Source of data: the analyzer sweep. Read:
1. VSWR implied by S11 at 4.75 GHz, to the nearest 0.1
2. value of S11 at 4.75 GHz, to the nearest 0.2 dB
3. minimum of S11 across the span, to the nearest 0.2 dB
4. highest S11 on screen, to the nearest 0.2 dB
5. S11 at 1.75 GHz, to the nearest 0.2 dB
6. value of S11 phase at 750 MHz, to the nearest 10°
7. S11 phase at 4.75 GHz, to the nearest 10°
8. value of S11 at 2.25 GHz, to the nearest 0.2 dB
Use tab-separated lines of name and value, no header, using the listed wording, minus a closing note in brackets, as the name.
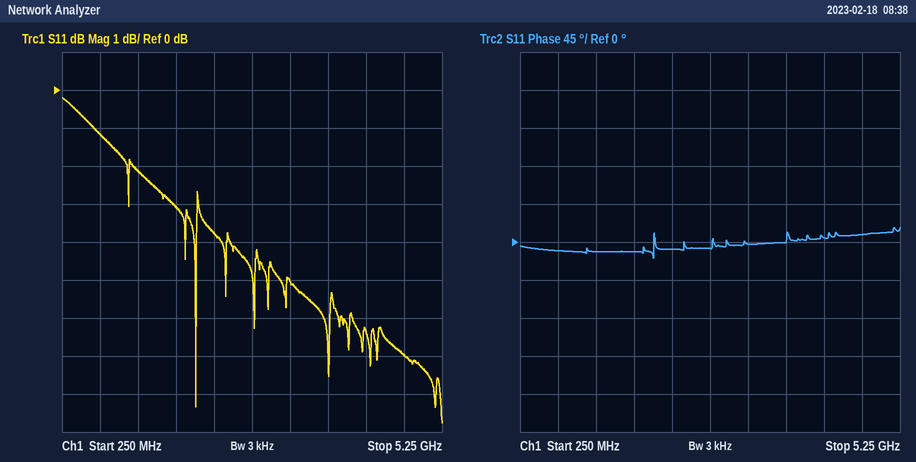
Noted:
VSWR implied by S11 at 4.75 GHz, to the nearest 0.1	2.6
value of S11 at 4.75 GHz, to the nearest 0.2 dB	-7.0 dB
minimum of S11 across the span, to the nearest 0.2 dB	-8.8 dB
highest S11 on screen, to the nearest 0.2 dB	-0.2 dB
S11 at 1.75 GHz, to the nearest 0.2 dB	-3.0 dB
value of S11 phase at 750 MHz, to the nearest 10°	-10°
S11 phase at 4.75 GHz, to the nearest 10°	10°
value of S11 at 2.25 GHz, to the nearest 0.2 dB	-3.8 dB
